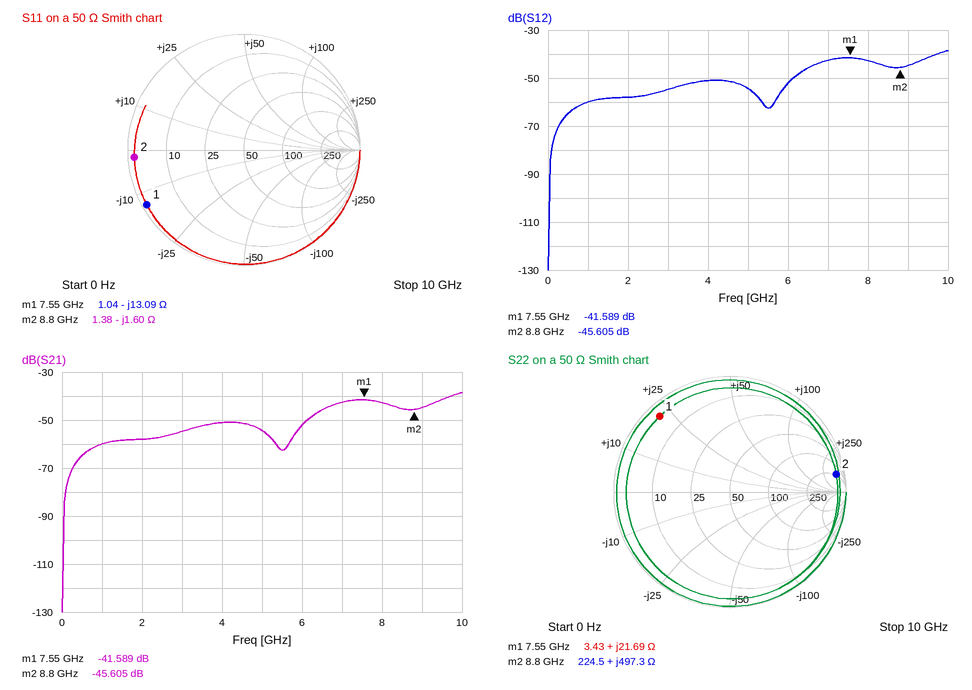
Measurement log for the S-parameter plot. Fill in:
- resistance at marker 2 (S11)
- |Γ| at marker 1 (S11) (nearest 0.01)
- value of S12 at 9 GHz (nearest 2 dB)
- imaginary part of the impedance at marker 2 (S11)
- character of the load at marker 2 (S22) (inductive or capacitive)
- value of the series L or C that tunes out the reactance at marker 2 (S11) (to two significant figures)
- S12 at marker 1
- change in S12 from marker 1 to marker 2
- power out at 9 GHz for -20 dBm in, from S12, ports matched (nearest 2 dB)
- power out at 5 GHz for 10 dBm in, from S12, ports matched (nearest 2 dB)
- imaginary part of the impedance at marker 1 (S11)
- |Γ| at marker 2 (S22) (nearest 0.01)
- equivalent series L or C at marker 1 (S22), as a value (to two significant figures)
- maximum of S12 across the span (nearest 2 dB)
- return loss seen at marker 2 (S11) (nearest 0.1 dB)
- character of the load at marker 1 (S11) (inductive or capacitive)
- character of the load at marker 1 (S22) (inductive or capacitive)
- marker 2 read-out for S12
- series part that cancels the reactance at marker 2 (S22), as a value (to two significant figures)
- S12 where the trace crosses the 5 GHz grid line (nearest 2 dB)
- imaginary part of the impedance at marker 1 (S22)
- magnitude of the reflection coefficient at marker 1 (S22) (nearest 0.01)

1.38 Ω
0.96
-44 dB
-1.60 Ω
inductive
29 pH
-41.589 dB
-4.016 dB
-64 dBm
-44 dBm
-13.09 Ω
0.93
460 pH
-38 dB
0.5 dB
capacitive
inductive
-45.605 dB
36 fF
-54 dB
+21.69 Ω
0.89
